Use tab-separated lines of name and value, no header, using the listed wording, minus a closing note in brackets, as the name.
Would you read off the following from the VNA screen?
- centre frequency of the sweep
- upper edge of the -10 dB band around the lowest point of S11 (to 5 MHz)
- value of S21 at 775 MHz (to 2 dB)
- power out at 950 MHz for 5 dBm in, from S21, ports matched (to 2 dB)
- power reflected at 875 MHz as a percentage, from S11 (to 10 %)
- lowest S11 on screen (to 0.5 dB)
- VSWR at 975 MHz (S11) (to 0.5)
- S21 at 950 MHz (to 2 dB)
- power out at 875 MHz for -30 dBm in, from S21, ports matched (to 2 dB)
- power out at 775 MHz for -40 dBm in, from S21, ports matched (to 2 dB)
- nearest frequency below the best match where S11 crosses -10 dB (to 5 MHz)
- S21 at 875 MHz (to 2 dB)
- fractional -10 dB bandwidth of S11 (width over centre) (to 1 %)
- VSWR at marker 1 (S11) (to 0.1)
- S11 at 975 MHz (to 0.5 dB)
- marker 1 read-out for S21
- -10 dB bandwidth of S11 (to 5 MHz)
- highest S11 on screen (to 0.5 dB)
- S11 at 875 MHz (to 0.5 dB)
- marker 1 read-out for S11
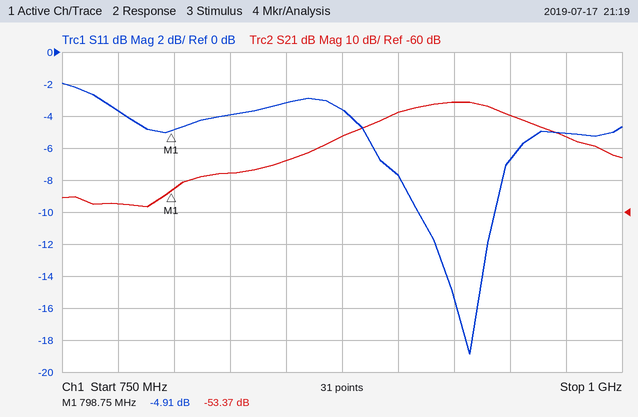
centre frequency of the sweep	875 MHz
upper edge of the -10 dB band around the lowest point of S11	945 MHz
value of S21 at 775 MHz	-58 dB
power out at 950 MHz for 5 dBm in, from S21, ports matched	-24 dBm
power reflected at 875 MHz as a percentage, from S11	40 %
lowest S11 on screen	-19.0 dB
VSWR at 975 MHz (S11)	3.5
S21 at 950 MHz	-30 dB
power out at 875 MHz for -30 dBm in, from S21, ports matched	-66 dBm
power out at 775 MHz for -40 dBm in, from S21, ports matched	-98 dBm
nearest frequency below the best match where S11 crosses -10 dB	910 MHz
S21 at 875 MHz	-36 dB
fractional -10 dB bandwidth of S11 (width over centre)	4 %
VSWR at marker 1 (S11)	3.6
S11 at 975 MHz	-5.0 dB
marker 1 read-out for S21	-53.37 dB
-10 dB bandwidth of S11	35 MHz
highest S11 on screen	-2.0 dB
S11 at 875 MHz	-3.5 dB
marker 1 read-out for S11	-4.91 dB
